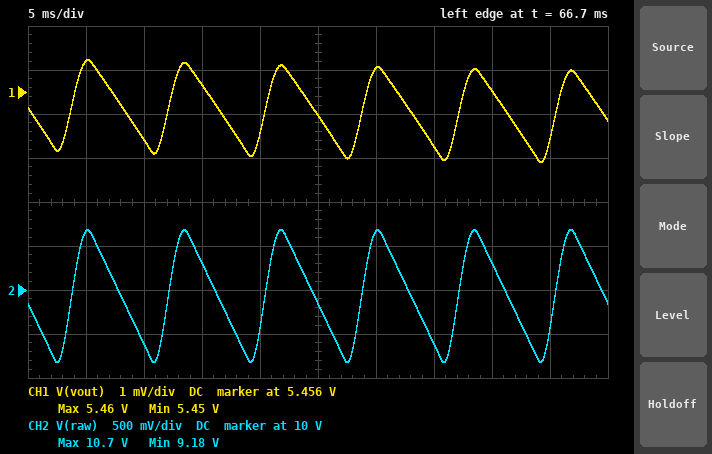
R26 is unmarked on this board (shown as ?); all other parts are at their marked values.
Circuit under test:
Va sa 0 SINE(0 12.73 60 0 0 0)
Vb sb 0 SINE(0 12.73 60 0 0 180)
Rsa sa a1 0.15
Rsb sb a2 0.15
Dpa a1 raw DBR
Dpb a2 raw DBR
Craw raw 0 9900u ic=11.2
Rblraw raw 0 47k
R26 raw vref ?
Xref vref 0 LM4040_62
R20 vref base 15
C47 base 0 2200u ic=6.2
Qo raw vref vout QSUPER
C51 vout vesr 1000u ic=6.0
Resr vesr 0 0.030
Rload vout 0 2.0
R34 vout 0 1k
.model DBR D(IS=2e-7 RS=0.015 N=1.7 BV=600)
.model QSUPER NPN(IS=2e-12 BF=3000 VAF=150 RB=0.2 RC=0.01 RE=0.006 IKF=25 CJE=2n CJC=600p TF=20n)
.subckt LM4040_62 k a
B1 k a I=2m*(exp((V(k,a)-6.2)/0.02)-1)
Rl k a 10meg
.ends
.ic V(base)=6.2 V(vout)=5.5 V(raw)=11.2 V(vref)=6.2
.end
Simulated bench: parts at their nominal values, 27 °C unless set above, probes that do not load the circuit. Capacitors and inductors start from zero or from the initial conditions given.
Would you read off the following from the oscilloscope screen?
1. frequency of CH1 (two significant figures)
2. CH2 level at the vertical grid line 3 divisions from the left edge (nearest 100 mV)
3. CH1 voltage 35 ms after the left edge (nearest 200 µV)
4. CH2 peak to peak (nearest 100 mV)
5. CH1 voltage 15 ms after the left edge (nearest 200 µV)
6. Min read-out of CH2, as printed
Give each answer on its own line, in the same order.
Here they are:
120 Hz
10.3 V
5.4548 V
1.5 V
5.4562 V
9.18 V
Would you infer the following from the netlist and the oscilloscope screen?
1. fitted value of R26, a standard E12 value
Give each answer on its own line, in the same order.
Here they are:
5.6 kΩ
